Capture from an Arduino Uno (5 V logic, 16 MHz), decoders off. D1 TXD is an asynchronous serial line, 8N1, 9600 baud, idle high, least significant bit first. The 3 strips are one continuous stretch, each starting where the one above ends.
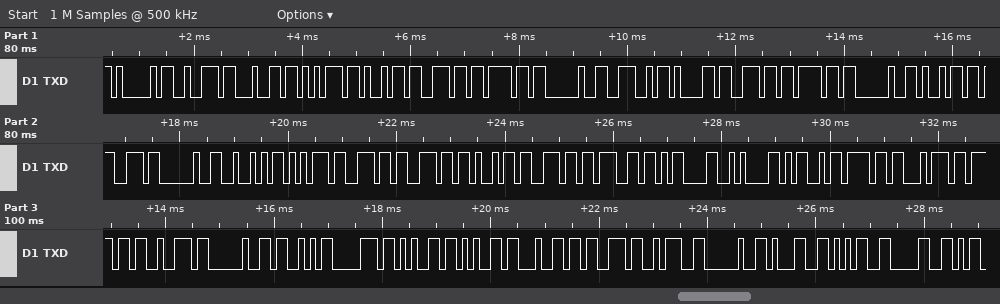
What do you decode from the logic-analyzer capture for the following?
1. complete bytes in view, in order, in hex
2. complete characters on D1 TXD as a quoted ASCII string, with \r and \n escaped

41 72 64 75 69 6E 6F 20 4E 61 6E 6F 20 69 73 20 52 75 6E 6E 69 6E 67 0D 0A 4D 6F 74 6F 72 20 53 70 65 65 64 73 3A 20 31 35 30
"Arduino Nano is Running\r\nMotor Speeds: 150"
